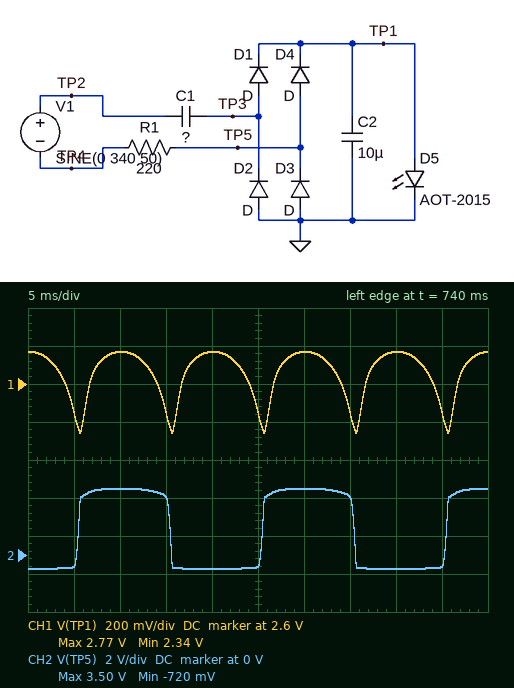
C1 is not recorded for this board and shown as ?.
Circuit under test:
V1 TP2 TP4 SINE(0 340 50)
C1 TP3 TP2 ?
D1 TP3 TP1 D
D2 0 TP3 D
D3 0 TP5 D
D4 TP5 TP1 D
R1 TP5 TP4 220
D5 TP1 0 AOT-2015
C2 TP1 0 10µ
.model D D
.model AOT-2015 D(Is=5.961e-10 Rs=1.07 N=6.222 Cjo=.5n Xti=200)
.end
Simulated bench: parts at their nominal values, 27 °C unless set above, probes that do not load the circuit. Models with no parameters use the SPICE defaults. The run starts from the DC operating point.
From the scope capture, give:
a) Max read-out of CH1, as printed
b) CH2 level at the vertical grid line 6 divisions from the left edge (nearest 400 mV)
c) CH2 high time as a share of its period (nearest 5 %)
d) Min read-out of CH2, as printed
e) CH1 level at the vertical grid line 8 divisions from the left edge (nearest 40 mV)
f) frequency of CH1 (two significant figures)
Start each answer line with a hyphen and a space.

- 2.77 V
- 3.6 V
- 50 %
- -720 mV
- 2.76 V
- 100 Hz
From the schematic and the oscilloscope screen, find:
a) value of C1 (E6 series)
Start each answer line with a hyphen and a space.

- 150 nF
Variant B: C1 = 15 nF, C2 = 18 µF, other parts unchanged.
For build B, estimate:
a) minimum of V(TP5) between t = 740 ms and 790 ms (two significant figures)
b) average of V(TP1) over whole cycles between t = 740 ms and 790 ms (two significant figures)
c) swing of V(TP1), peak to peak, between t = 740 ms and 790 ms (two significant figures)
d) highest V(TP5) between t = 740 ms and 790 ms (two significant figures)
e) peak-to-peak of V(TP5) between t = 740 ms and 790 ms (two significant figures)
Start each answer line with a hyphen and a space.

- -670 mV
- 2.3 V
- 110 mV
- 3.0 V
- 3.7 V
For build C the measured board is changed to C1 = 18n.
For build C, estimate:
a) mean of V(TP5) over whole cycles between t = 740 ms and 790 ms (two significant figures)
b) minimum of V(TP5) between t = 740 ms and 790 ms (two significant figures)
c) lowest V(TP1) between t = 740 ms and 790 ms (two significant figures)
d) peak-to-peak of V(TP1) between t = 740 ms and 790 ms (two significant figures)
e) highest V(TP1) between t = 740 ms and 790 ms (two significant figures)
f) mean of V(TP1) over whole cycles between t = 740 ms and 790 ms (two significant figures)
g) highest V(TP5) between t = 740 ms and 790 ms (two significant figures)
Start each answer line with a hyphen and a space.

- 1.2 V
- -670 mV
- 2.2 V
- 190 mV
- 2.4 V
- 2.3 V
- 3.1 V
